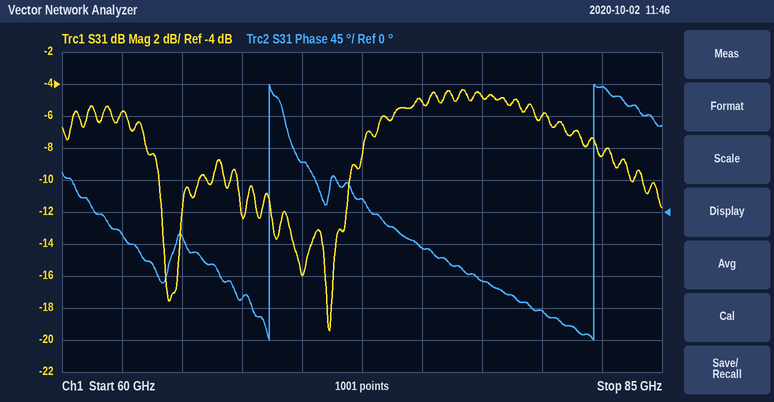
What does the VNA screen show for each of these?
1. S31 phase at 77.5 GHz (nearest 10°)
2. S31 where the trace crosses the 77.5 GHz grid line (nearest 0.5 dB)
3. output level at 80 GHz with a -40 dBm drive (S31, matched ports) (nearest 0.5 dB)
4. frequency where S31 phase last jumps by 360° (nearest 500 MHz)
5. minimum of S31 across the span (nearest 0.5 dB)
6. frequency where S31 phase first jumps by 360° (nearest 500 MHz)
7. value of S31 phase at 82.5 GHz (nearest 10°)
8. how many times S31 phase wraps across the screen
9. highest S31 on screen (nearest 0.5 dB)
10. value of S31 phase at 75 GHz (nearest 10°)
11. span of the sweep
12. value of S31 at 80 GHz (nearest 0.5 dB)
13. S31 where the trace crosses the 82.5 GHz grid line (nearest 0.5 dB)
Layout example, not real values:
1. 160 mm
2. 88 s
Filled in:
1. -100°
2. -5.0 dB
3. -46.0 dBm
4. 82.0 GHz
5. -19.5 dB
6. 68.5 GHz
7. 180°
8. 2
9. -4.5 dB
10. -50°
11. 25 GHz
12. -6.0 dB
13. -8.5 dB
